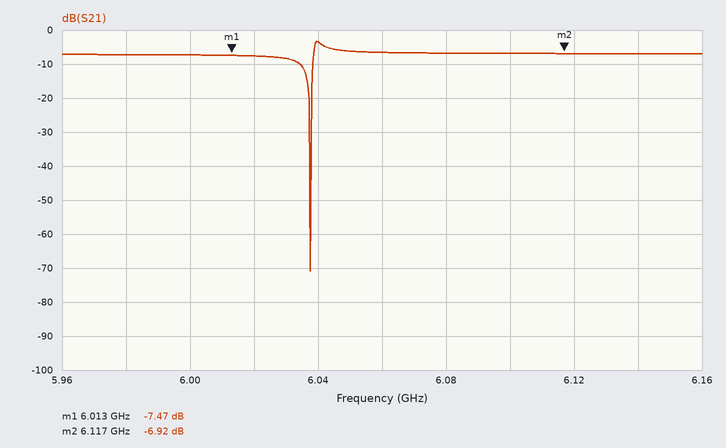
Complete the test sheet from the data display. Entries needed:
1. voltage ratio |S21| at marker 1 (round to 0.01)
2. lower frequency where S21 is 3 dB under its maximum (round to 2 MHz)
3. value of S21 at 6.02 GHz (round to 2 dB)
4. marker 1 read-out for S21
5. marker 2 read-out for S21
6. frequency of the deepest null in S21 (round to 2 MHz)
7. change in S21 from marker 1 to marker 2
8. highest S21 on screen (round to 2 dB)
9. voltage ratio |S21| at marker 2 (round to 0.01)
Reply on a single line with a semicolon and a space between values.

0.42; 6.038 GHz; -8 dB; -7.47 dB; -6.92 dB; 6.038 GHz; 0.55 dB; -4 dB; 0.45
